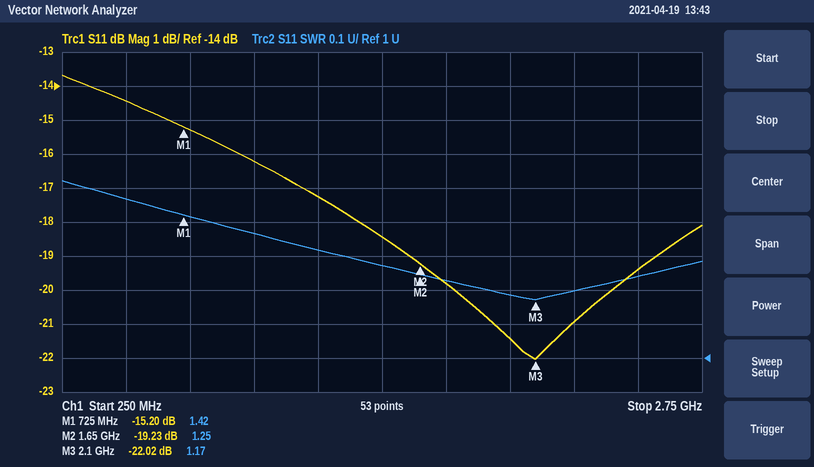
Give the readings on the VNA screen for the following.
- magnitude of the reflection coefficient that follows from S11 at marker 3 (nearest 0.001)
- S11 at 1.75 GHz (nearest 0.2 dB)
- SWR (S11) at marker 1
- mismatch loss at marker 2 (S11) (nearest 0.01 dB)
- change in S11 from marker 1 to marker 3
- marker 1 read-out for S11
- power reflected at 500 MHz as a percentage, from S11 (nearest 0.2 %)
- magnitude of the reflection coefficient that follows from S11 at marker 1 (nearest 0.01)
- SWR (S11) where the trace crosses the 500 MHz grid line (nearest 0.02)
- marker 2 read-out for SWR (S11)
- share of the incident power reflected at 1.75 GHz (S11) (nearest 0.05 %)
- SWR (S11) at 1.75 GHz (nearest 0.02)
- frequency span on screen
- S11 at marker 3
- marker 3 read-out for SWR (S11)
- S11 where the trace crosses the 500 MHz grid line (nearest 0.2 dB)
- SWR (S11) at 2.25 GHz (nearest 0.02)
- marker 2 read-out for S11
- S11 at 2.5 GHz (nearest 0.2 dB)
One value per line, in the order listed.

0.079
-19.8 dB
1.42
0.05 dB
-6.82 dB
-15.20 dB
3.6 %
0.17
1.46
1.25
1.05 %
1.22
2.5 GHz
-22.02 dB
1.17
-14.4 dB
1.20
-19.23 dB
-19.4 dB
